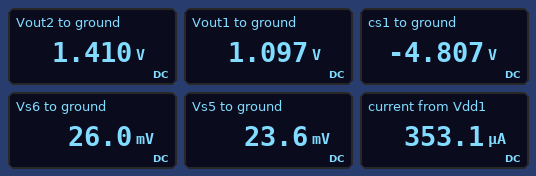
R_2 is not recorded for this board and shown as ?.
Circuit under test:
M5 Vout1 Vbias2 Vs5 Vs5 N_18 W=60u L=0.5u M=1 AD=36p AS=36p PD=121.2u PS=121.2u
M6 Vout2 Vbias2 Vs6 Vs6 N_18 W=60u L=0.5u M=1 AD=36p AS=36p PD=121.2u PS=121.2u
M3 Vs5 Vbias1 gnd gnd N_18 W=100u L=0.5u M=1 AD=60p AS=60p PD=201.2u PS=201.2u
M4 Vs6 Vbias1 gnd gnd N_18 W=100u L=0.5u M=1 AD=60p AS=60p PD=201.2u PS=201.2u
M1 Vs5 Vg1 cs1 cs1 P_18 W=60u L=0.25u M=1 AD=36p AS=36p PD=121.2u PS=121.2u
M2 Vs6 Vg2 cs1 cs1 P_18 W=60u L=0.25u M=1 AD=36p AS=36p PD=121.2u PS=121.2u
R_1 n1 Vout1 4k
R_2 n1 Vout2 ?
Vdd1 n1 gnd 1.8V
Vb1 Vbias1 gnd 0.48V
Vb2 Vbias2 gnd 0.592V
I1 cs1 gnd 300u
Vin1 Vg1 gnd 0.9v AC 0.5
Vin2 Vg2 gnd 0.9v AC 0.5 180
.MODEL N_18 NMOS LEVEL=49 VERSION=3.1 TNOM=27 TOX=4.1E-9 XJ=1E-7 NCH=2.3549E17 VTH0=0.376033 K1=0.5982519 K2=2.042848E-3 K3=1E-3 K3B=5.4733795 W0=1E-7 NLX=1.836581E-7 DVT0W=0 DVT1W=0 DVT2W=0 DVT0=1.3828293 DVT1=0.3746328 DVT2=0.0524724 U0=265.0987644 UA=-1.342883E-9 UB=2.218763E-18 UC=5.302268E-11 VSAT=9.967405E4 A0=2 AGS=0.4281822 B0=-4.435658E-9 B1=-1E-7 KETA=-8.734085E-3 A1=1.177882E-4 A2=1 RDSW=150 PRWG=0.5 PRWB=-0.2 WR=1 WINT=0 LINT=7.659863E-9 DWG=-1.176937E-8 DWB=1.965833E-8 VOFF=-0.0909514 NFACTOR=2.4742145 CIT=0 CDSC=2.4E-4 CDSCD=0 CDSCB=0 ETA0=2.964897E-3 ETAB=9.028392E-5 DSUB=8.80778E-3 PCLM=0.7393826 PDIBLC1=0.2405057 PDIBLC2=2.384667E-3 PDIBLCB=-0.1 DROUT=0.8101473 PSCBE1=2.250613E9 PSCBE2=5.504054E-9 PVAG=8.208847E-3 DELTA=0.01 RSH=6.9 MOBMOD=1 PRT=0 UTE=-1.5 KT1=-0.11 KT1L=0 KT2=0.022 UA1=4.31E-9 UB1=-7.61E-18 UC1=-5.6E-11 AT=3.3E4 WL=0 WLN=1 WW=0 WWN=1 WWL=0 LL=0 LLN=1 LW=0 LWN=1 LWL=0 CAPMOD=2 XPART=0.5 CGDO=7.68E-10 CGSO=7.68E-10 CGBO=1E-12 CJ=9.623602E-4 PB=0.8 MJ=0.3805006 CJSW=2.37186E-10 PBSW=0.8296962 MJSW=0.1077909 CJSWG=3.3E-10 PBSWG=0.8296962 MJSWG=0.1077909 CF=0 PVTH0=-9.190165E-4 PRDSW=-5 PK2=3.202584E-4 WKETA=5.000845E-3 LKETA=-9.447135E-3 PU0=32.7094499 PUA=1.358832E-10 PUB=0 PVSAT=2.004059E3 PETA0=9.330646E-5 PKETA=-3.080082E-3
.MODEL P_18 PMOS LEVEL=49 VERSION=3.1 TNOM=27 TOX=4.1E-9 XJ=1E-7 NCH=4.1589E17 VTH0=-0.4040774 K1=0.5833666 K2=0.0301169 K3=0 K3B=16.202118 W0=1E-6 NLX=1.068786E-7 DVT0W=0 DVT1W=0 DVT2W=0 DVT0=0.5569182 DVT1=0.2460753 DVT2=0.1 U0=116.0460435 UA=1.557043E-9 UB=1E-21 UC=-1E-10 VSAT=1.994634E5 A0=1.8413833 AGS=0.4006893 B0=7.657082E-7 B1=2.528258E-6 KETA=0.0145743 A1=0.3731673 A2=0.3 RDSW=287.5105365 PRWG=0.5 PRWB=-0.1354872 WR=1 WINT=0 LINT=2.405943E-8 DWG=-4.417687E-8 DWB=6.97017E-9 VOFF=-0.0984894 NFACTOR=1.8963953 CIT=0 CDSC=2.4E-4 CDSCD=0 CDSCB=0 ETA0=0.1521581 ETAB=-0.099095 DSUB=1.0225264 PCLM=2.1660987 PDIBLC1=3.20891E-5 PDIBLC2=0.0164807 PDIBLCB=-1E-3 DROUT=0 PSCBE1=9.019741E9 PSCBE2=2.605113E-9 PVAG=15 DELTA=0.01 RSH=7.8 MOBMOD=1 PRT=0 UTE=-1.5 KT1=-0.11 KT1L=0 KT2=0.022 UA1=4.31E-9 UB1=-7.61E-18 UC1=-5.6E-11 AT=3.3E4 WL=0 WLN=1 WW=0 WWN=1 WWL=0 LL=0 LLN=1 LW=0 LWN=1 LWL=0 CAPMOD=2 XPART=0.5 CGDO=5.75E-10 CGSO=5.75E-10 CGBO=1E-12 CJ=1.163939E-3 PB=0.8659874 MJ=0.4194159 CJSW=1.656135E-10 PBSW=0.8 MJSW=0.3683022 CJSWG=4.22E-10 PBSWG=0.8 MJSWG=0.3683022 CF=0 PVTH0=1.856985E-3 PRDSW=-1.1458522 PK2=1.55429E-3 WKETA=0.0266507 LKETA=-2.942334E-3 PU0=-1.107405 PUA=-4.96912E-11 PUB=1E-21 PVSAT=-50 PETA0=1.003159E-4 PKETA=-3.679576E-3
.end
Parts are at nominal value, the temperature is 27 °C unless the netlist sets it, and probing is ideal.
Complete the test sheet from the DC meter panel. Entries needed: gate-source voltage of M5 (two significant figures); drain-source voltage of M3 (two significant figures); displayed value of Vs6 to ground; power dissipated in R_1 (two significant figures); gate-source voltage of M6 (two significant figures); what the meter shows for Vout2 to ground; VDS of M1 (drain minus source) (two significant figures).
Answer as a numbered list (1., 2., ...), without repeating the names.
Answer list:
1. 570 mV
2. 24 mV
3. 26.0 mV
4. 120 µW
5. 570 mV
6. 1.410 V
7. 4.8 V
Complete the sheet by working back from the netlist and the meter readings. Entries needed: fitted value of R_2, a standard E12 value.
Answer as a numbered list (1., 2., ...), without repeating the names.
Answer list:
1. 2.2 kΩ
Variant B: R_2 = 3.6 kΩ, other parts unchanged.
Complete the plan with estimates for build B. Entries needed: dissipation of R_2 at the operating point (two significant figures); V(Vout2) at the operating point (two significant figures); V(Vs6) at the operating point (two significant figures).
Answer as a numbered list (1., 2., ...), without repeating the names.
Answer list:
1. 110 µW
2. 1.2 V
3. 24 mV
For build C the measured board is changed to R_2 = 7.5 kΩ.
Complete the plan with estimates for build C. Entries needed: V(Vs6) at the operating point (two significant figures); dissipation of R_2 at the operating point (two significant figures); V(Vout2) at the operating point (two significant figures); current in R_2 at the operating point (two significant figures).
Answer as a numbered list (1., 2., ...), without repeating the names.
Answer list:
1. 19 mV
2. 220 µW
3. 510 mV
4. 170 µA
